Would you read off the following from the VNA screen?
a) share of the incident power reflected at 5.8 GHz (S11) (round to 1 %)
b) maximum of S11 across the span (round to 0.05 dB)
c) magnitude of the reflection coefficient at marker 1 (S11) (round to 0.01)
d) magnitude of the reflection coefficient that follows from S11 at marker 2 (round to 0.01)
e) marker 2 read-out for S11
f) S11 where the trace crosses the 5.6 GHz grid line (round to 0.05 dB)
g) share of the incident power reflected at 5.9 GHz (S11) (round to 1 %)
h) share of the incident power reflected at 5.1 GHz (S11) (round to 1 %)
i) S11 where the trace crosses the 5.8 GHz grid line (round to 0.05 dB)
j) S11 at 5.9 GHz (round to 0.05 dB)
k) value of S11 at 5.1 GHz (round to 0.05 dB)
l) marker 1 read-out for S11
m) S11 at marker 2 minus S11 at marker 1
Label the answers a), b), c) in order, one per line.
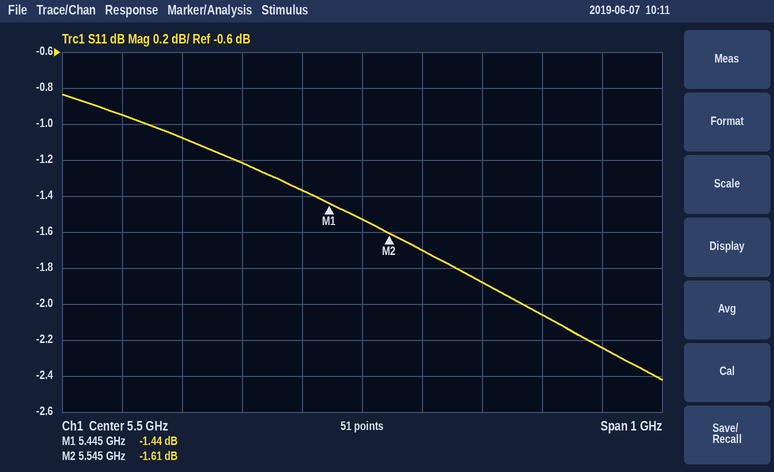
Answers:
a) 62 %
b) -0.85 dB
c) 0.85
d) 0.83
e) -1.61 dB
f) -1.70 dB
g) 60 %
h) 80 %
i) -2.05 dB
j) -2.25 dB
k) -0.95 dB
l) -1.44 dB
m) -0.17 dB
